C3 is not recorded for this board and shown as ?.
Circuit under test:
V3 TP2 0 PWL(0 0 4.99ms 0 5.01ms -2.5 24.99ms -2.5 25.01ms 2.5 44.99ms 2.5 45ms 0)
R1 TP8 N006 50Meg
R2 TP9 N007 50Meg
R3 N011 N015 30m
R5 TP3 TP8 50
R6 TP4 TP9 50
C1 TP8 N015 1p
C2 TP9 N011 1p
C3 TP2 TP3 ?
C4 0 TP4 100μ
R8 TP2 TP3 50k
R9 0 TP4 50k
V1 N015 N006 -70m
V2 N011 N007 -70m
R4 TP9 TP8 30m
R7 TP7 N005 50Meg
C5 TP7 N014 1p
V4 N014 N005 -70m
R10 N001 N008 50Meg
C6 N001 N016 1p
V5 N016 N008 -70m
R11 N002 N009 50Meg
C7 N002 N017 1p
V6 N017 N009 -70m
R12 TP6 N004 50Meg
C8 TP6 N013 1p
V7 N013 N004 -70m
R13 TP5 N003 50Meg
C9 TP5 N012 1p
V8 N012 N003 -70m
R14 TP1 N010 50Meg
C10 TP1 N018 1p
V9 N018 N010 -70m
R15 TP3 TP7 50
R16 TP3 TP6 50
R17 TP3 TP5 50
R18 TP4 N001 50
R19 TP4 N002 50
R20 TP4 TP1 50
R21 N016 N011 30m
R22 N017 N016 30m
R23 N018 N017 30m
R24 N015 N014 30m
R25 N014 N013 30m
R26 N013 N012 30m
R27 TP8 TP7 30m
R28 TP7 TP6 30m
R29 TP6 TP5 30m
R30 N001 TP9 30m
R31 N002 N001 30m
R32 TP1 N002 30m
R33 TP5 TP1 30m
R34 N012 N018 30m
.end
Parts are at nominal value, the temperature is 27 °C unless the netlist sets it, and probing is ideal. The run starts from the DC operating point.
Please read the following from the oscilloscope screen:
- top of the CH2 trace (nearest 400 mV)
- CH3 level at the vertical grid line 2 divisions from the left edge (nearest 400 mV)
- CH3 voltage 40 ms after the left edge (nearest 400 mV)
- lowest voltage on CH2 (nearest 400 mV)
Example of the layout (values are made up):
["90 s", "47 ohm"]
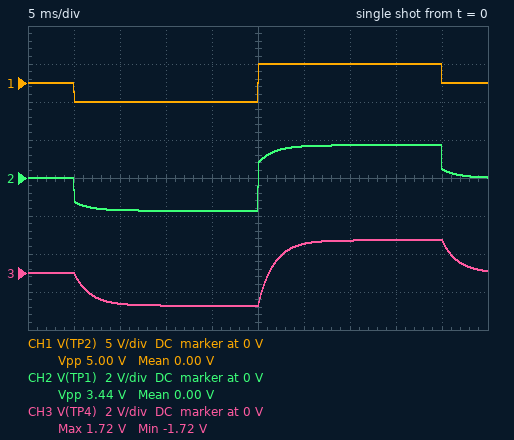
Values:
["1.6 V", "-1.6 V", "1.6 V", "-1.6 V"]
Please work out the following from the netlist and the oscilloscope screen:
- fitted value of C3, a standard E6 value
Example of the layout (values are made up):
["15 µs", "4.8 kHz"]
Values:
["220 µF"]
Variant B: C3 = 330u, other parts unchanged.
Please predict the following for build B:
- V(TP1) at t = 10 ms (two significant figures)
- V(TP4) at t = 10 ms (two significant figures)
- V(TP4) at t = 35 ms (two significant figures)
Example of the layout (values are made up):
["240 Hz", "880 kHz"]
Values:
["-1.9 V", "-1.8 V", "1.9 V"]
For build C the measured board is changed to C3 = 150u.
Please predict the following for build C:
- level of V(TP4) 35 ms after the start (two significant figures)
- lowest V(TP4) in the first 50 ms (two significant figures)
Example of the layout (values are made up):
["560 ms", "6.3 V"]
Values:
["1.5 V", "-1.5 V"]
